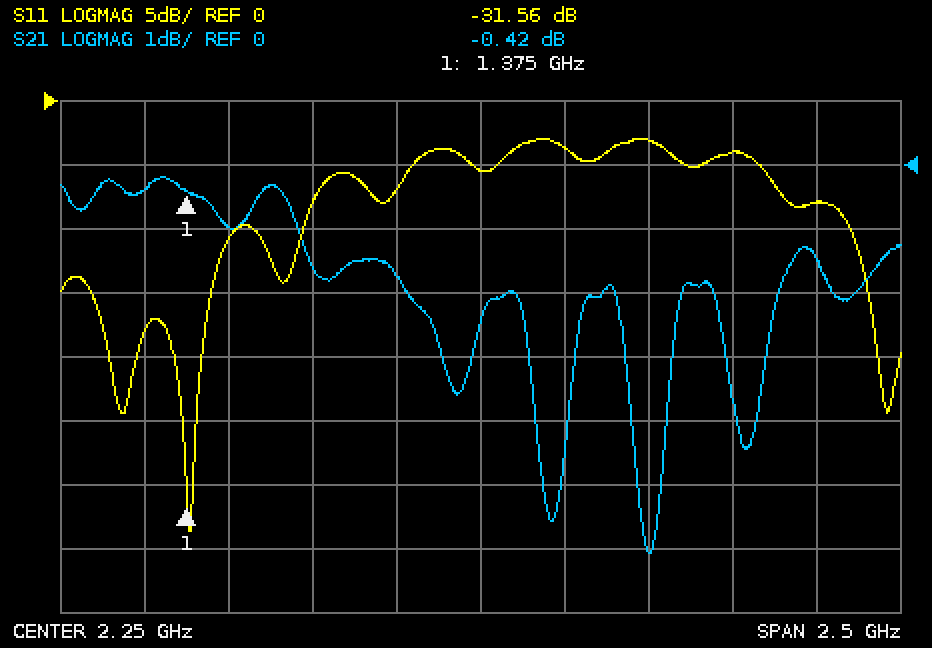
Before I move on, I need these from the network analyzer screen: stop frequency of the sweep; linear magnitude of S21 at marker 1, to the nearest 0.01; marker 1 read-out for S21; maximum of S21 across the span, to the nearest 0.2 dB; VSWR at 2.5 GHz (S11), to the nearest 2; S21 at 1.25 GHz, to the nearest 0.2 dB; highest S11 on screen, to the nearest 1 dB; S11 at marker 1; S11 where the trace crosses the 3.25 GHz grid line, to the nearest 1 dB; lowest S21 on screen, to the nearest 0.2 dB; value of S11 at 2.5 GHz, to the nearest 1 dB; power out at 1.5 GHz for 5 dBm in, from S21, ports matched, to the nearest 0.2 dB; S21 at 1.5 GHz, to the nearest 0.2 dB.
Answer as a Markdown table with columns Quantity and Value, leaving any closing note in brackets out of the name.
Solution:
| Quantity | Value |
|---|---|
| stop frequency of the sweep | 3.5 GHz |
| linear magnitude of S21 at marker 1, to the nearest 0.01 | 0.95 |
| marker 1 read-out for S21 | -0.42 dB |
| maximum of S21 across the span, to the nearest 0.2 dB | -0.2 dB |
| VSWR at 2.5 GHz (S11), to the nearest 2 | 4 |
| S21 at 1.25 GHz, to the nearest 0.2 dB | -0.4 dB |
| highest S11 on screen, to the nearest 1 dB | -3 dB |
| S11 at marker 1 | -31.56 dB |
| S11 where the trace crosses the 3.25 GHz grid line, to the nearest 1 dB | -8 dB |
| lowest S21 on screen, to the nearest 0.2 dB | -6.0 dB |
| value of S11 at 2.5 GHz, to the nearest 1 dB | -4 dB |
| power out at 1.5 GHz for 5 dBm in, from S21, ports matched, to the nearest 0.2 dB | 4.0 dBm |
| S21 at 1.5 GHz, to the nearest 0.2 dB | -1.0 dB |
